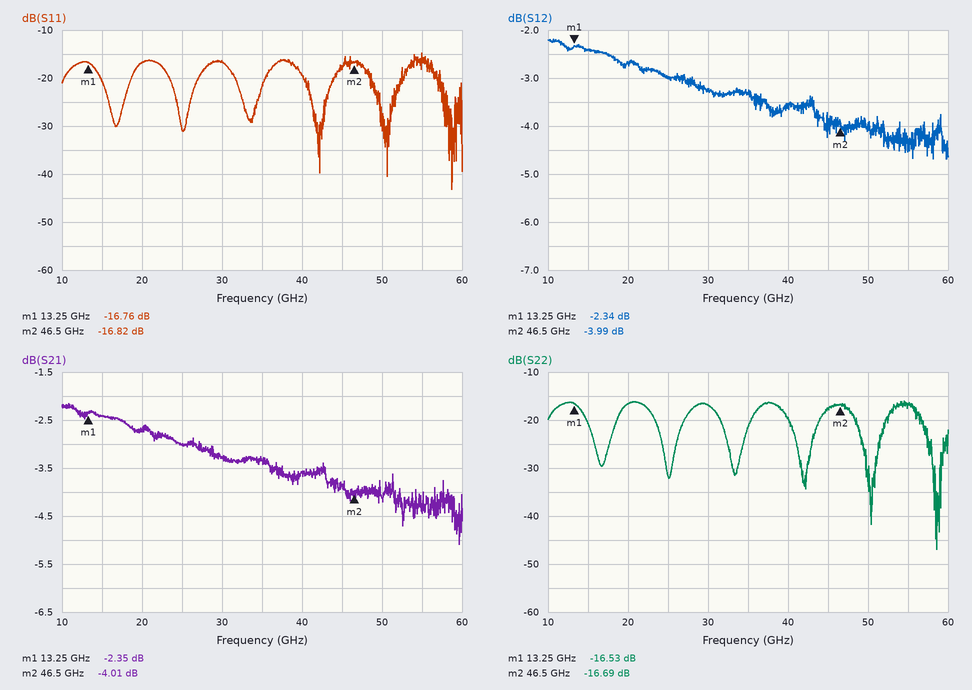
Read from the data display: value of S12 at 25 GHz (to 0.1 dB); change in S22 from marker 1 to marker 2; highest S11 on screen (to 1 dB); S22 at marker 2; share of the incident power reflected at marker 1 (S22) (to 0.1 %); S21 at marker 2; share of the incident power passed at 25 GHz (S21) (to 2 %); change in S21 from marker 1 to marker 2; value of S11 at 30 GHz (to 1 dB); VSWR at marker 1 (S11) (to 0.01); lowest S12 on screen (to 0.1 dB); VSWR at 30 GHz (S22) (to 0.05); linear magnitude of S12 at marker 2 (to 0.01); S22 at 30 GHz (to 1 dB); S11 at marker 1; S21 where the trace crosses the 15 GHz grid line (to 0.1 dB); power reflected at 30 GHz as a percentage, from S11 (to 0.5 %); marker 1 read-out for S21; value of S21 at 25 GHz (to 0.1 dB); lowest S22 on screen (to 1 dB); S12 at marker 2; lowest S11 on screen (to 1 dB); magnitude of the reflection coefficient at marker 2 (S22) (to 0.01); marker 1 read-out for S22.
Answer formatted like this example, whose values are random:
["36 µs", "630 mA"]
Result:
["-3.0 dB", "-0.16 dB", "-15 dB", "-16.69 dB", "2.2 %", "-4.01 dB", "50 %", "-1.66 dB", "-17 dB", "1.34", "-4.7 dB", "1.35", "0.63", "-17 dB", "-16.76 dB", "-2.4 dB", "2.0 %", "-2.35 dB", "-3.0 dB", "-47 dB", "-3.99 dB", "-43 dB", "0.15", "-16.53 dB"]
